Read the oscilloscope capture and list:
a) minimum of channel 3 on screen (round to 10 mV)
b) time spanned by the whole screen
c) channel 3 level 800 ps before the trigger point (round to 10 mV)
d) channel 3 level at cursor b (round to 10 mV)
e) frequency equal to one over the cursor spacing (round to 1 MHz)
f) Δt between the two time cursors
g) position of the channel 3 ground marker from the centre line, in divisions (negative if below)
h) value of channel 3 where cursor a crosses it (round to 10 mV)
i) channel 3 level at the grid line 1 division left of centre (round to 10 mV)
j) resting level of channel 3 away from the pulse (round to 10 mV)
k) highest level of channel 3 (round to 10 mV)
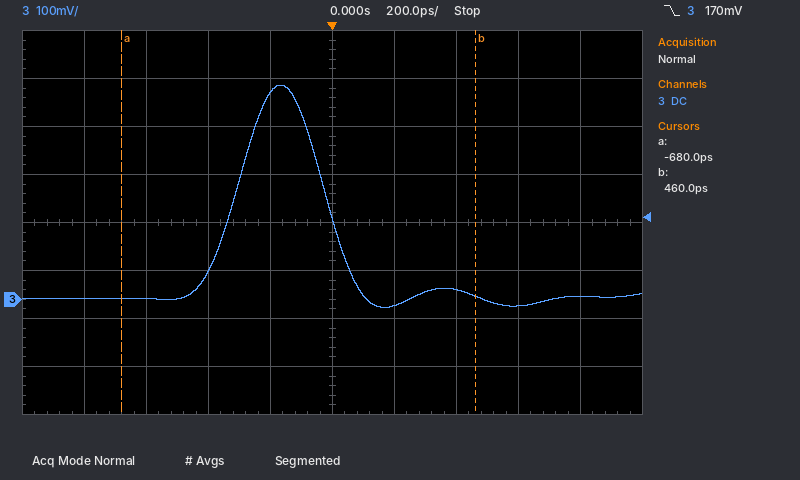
-20 mV
2 ns
0 mV
10 mV
877 MHz
1.14 ns
-1.6 div
0 mV
430 mV
0 mV
450 mV
